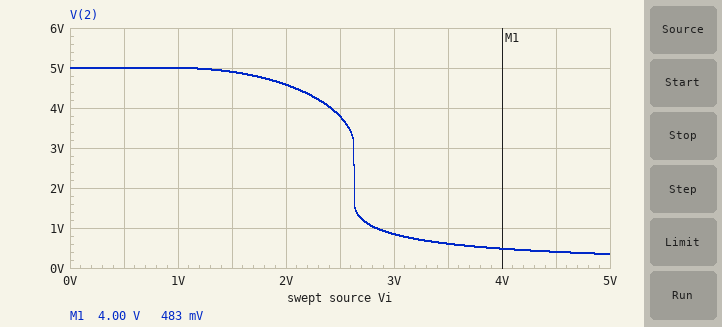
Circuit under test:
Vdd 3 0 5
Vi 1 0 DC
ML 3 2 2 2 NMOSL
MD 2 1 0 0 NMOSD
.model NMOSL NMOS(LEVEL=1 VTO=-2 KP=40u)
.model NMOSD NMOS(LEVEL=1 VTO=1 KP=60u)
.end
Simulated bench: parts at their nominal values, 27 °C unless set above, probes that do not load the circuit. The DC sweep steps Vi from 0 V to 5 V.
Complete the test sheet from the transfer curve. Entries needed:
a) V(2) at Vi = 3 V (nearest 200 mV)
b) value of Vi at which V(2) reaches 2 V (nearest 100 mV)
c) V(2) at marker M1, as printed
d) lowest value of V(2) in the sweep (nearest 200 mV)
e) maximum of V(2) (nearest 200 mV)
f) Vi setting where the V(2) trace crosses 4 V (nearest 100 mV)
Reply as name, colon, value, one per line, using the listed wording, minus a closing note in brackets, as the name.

V(2) at Vi = 3 V: 800 mV
value of Vi at which V(2) reaches 2 V: 2.6 V
V(2) at marker M1, as printed: 483 mV
lowest value of V(2) in the sweep: 400 mV
maximum of V(2): 5.0 V
Vi setting where the V(2) trace crosses 4 V: 2.4 V
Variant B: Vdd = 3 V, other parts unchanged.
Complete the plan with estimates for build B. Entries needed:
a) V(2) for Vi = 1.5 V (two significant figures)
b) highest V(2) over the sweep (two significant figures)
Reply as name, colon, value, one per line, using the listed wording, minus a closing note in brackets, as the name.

V(2) for Vi = 1.5 V: 2.9 V
highest V(2) over the sweep: 3.0 V
